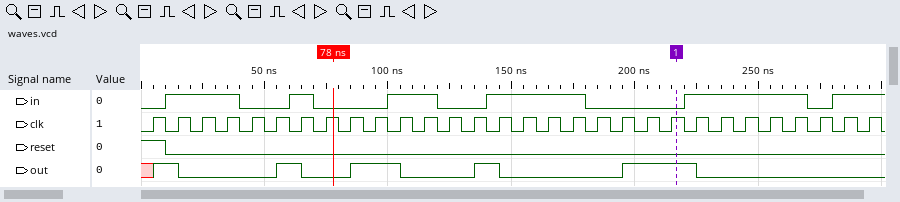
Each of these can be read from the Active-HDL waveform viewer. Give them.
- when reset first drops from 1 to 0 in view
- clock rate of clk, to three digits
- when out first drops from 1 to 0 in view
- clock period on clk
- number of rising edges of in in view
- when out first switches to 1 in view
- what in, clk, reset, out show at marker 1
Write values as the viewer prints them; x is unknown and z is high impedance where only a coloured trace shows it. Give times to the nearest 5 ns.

10 ns
100 MHz
15 ns
10 ns
6
5 ns
in=0, clk=1, reset=0, out=1
